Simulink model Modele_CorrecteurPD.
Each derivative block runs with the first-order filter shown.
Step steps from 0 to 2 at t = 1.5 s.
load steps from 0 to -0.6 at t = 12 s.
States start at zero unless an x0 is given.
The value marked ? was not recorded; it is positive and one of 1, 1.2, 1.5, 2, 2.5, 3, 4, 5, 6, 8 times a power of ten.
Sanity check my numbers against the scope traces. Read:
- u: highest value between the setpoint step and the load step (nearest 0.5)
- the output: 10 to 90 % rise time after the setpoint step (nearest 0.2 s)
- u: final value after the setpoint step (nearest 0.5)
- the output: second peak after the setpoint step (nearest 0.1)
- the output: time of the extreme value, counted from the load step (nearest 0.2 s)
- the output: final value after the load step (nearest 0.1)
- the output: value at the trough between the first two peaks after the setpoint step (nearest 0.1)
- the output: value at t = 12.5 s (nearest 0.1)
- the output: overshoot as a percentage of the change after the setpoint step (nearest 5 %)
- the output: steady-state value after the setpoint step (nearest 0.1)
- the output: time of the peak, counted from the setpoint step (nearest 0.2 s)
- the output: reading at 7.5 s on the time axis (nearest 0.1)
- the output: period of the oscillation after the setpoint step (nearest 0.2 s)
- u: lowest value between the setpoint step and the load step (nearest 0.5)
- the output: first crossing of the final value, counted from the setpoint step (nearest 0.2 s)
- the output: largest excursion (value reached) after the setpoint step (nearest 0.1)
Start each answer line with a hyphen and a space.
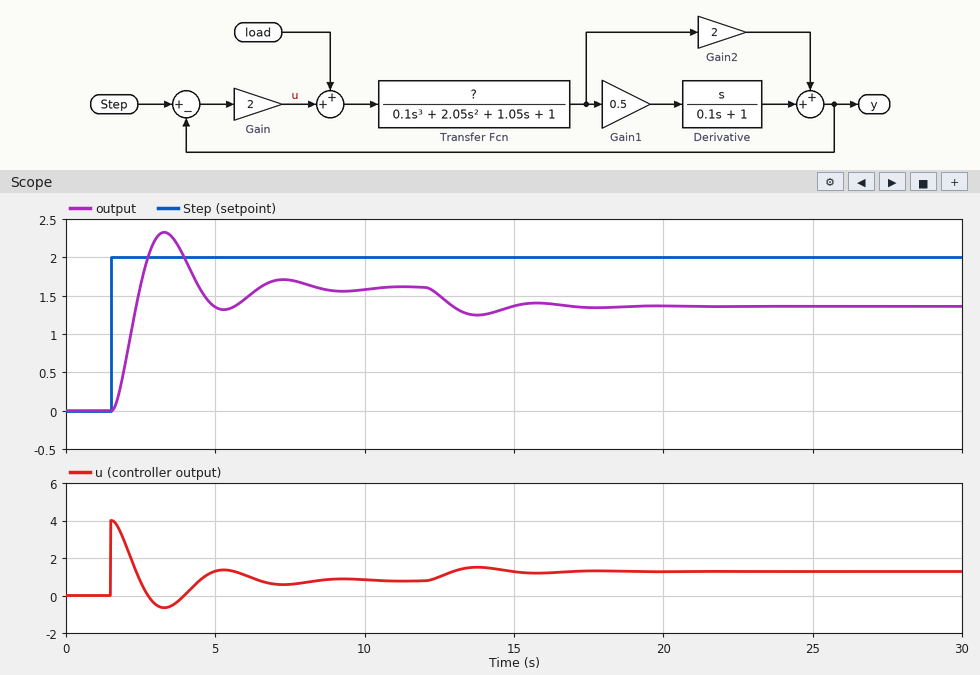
- 4.0
- 0.6 s
- 1.0
- 1.7
- 1.8 s
- 1.4
- 1.3
- 1.5
- 45 %
- 1.6
- 1.8 s
- 1.7
- 4.0 s
- -0.5
- 1.0 s
- 2.3
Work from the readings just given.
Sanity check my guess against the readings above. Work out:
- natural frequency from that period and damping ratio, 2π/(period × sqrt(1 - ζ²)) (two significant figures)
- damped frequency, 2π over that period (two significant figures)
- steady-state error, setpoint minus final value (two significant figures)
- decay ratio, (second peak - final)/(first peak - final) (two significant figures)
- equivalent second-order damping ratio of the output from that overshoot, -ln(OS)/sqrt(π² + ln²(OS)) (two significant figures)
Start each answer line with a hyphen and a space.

- 1.6 rad/s
- 1.6 rad/s
- 0.40
- 0.14
- 0.25
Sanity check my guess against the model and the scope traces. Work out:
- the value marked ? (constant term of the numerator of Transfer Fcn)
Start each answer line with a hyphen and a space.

- 1
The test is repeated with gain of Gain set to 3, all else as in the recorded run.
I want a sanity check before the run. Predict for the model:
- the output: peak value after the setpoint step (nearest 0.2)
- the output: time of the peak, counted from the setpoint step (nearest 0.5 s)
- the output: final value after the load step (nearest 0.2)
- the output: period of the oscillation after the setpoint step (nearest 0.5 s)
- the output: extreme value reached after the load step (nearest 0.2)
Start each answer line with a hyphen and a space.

- 2.6
- 1.5 s
- 1.6
- 3.5 s
- 1.4
